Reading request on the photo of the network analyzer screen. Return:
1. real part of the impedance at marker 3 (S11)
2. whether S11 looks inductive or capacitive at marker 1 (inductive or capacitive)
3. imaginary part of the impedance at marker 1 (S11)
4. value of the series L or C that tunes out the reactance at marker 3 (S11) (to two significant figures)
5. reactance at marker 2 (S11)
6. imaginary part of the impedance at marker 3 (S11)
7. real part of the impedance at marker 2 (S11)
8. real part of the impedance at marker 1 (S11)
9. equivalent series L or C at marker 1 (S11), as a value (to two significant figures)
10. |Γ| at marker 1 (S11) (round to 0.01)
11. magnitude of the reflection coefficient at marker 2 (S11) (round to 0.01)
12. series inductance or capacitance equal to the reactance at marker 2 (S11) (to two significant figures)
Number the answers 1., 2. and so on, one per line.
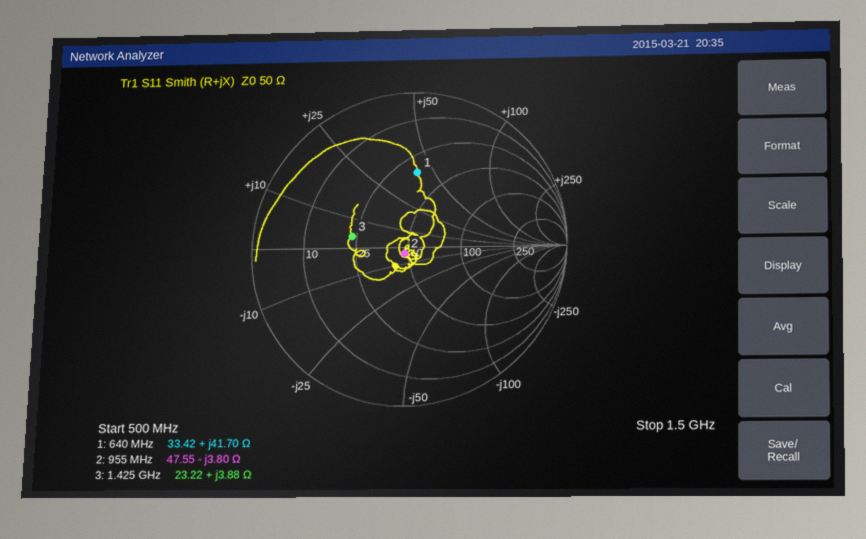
1. 23.22 Ω
2. inductive
3. +41.70 Ω
4. 29 pF
5. -3.80 Ω
6. +3.88 Ω
7. 47.55 Ω
8. 33.42 Ω
9. 10 nH
10. 0.48
11. 0.05
12. 44 pF
